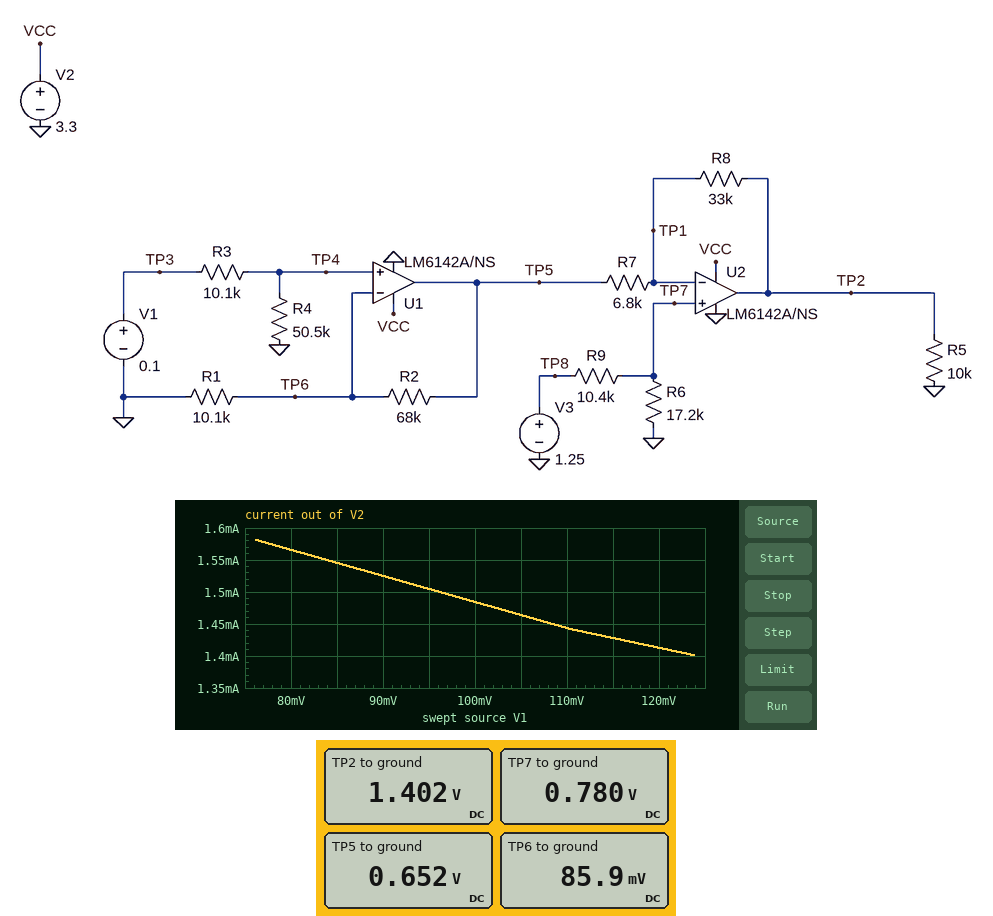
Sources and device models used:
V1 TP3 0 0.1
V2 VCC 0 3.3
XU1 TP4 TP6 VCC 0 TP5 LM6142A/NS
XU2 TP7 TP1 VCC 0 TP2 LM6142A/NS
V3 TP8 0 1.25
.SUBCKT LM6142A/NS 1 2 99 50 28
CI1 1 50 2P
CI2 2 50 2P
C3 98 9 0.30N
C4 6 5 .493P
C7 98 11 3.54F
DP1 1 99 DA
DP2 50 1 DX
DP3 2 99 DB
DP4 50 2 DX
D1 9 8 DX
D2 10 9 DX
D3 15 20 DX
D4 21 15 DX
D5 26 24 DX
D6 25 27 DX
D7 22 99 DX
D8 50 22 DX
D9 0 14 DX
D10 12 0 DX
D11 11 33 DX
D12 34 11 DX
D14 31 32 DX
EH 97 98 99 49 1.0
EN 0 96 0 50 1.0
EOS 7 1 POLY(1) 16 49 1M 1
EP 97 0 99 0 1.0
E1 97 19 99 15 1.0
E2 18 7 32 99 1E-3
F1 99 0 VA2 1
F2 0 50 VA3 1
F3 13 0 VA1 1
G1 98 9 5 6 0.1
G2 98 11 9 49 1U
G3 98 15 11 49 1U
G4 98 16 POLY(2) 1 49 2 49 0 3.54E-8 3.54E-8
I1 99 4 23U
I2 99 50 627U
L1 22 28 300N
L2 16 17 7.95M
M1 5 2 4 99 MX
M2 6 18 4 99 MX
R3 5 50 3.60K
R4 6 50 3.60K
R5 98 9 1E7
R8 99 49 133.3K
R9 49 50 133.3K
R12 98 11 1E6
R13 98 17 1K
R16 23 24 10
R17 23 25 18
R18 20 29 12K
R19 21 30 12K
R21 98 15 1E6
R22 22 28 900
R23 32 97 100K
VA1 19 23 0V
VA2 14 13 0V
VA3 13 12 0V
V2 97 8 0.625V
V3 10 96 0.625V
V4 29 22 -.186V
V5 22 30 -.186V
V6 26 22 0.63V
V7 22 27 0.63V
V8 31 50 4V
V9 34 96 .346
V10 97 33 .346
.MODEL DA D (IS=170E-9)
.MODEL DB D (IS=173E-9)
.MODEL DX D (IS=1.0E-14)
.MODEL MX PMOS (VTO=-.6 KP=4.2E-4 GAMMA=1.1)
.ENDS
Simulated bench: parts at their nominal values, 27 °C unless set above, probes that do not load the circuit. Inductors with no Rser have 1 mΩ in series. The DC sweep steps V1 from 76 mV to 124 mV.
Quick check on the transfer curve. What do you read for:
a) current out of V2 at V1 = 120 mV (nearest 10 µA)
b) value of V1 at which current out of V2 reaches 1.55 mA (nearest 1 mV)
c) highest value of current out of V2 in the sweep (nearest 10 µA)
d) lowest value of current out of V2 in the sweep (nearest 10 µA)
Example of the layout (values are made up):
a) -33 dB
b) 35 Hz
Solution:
a) 1.41 mA
b) 84 mV
c) 1.58 mA
d) 1.40 mA
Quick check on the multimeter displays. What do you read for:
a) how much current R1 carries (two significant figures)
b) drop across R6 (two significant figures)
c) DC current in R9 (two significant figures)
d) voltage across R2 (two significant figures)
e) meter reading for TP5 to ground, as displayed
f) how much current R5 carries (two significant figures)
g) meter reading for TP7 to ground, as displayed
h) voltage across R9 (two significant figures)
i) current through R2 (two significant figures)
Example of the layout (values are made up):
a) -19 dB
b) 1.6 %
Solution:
a) 8.5 µA
b) 780 mV
c) 45 µA
d) 570 mV
e) 0.652 V
f) 140 µA
g) 0.780 V
h) 470 mV
i) 8.3 µA
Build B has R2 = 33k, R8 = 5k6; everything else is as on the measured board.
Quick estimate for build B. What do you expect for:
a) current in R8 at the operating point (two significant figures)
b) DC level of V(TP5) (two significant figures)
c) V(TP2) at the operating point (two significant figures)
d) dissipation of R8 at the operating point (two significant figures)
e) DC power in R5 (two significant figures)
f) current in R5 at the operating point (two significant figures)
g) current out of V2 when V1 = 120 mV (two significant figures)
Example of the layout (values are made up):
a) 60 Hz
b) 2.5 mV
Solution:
a) 62 µA
b) 360 mV
c) 1.1 V
d) 21 µW
e) 130 µW
f) 110 µA
g) 1.5 mA
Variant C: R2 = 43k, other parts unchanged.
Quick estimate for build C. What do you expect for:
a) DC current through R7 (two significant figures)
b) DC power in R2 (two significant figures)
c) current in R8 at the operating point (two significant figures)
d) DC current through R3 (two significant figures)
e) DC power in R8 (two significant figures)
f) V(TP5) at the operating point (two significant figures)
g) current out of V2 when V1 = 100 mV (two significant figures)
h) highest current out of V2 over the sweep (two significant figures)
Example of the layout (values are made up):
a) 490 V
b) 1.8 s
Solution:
a) 50 µA
b) 3.0 µW
c) 49 µA
d) 1.5 µA
e) 81 µW
f) 440 mV
g) 1.6 mA
h) 1.7 mA
